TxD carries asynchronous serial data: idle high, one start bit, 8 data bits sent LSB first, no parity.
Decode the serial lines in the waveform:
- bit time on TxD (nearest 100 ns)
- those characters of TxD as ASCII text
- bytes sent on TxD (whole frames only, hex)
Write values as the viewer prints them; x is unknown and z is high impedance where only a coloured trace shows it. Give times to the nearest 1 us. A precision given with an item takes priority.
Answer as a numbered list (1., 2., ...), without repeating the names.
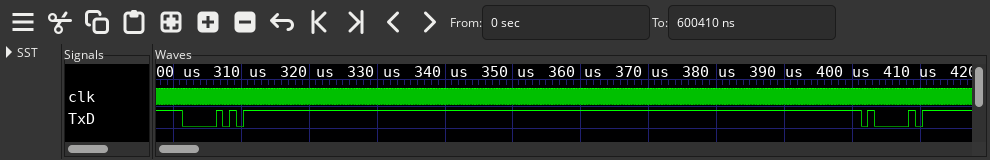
1. 1000 ns
2. "PA"
3. 50, 41
